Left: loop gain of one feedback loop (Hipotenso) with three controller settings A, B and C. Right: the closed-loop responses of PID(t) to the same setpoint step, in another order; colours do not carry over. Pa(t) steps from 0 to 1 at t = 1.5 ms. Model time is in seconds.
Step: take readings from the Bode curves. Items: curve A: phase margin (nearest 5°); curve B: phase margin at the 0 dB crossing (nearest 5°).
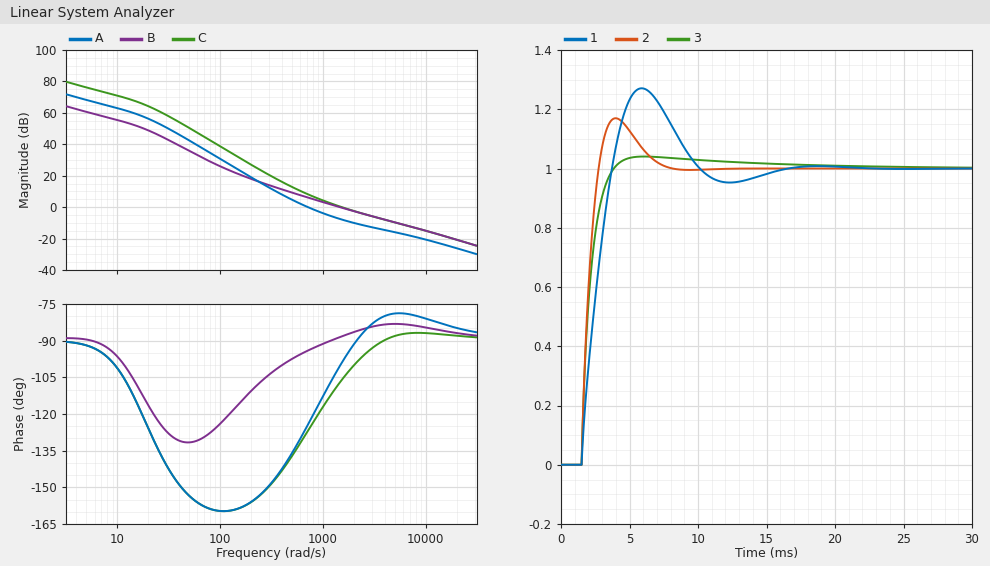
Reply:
55°
90°
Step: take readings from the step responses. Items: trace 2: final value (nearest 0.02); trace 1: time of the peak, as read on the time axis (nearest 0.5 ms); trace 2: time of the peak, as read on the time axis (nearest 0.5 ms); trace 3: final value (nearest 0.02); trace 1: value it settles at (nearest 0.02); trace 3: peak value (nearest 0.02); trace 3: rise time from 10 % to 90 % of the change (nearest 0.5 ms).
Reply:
1.00
6.0 ms
4.0 ms
1.00
1.00
1.04
1.5 ms
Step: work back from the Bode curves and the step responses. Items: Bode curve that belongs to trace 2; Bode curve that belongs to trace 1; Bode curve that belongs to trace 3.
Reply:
C
A
B
